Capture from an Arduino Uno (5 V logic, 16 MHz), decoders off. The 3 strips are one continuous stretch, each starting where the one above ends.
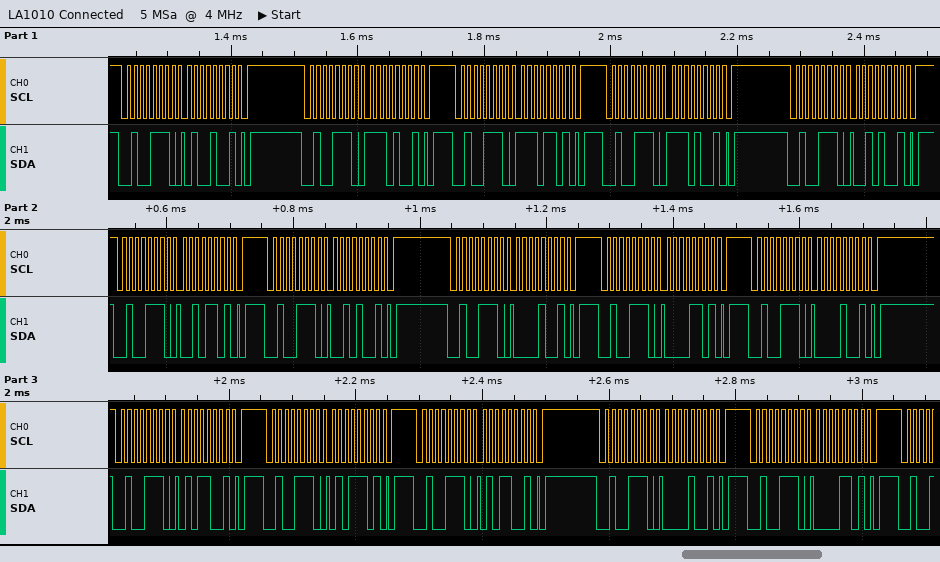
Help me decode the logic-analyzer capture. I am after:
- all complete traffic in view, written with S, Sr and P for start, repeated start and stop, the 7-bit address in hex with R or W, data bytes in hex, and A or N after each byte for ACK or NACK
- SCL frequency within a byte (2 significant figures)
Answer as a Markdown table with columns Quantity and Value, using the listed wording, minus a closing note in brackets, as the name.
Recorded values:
| Quantity | Value |
|---|---|
| all complete traffic in view, written with S, Sr and P for start, repeated start and stop, the 7-bit address in hex with R or W, data bytes in hex, and A or N after each byte for ACK or NACK | S 27W A 49 A P S 27W A E9 A P S 27W A ED A P S 27W A E9 A P S 27W A 29 A P S 27W A 2D A P S 27W A 29 A P S 27W A 09 A P S 27W A 0D A P S 27W A 09 A P S 27W A 59 A P S 27W A 5D A P S 27W A 59 A P S 27W A 09 A P S 27W A 0D A P |
| SCL frequency within a byte | 100 kHz |
